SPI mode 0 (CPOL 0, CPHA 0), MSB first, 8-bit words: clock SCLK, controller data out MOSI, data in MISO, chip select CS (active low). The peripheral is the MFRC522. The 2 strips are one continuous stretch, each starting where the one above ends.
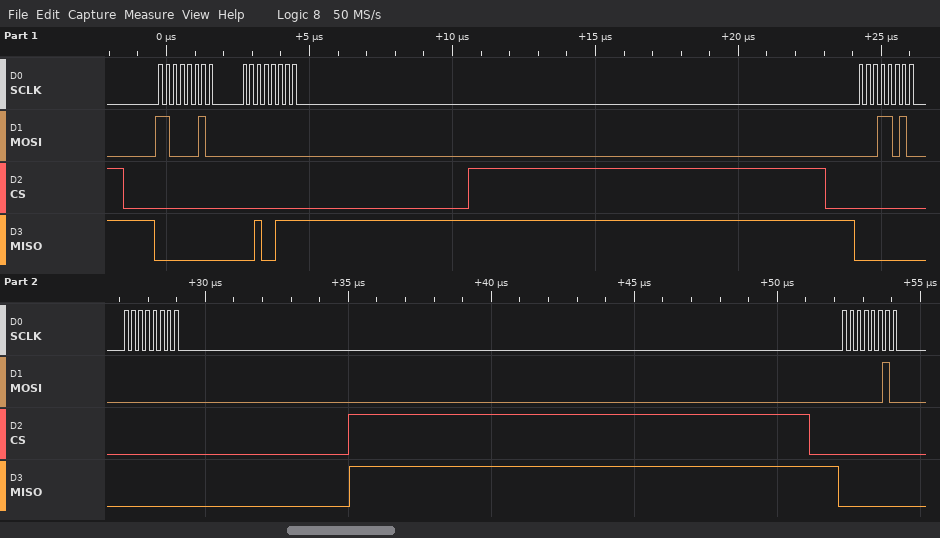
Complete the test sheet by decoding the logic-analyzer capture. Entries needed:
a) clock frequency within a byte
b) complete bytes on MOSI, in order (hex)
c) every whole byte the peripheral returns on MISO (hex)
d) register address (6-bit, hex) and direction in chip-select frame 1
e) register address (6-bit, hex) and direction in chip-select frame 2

4 MHz
0xC2 0x00 0x1A 0x00 0x02
0x00 0x27 0x00 0x00 0x00
0x21 read
0x0D write
